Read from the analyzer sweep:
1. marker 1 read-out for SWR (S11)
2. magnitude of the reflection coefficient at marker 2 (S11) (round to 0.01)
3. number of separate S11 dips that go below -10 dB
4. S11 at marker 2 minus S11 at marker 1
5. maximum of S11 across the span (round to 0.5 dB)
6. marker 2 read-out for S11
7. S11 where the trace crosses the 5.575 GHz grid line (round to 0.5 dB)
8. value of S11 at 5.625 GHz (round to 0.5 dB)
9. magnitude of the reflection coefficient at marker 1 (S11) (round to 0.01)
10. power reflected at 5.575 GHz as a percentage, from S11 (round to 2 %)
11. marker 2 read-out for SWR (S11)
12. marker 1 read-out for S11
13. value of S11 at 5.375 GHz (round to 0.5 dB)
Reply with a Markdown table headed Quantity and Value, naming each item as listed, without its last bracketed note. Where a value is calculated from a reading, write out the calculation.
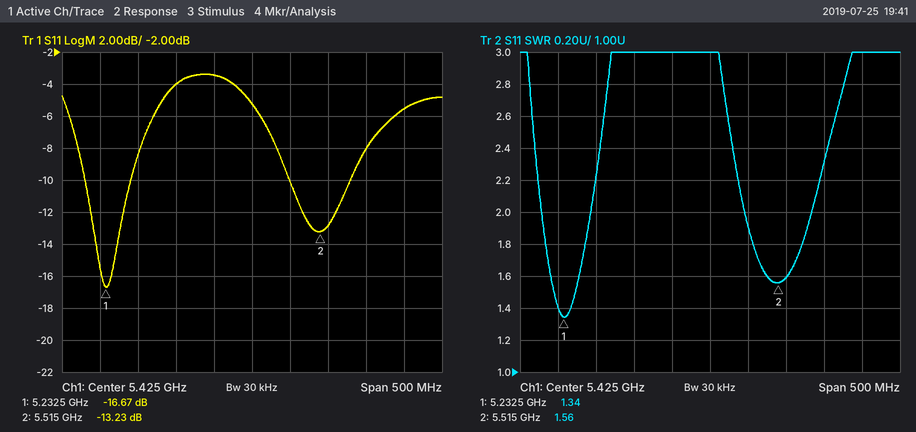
| Quantity | Value |
|---|---|
| marker 1 read-out for SWR | 1.34 |
| magnitude of the reflection coefficient at marker 2 (S11) | 10^(-13.23/20) ≈ 0.22 |
| number of separate S11 dips that go below -10 dB | 2 |
| S11 at marker 2 minus S11 at marker 1 | -13.23 − (-16.67) = 3.44 dB |
| maximum of S11 across the span | -3.5 dB |
| marker 2 read-out for S11 | -13.23 dB |
| S11 where the trace crosses the 5.575 GHz grid line | -8.0 dB |
| value of S11 at 5.625 GHz | -5.5 dB |
| magnitude of the reflection coefficient at marker 1 (S11) | 10^(-16.67/20) ≈ 0.15 |
| power reflected at 5.575 GHz as a percentage, from S11 | 10^(-8/10) ≈ 16 % |
| marker 2 read-out for SWR | 1.56 |
| marker 1 read-out for S11 | -16.67 dB |
| value of S11 at 5.375 GHz | -3.5 dB |
